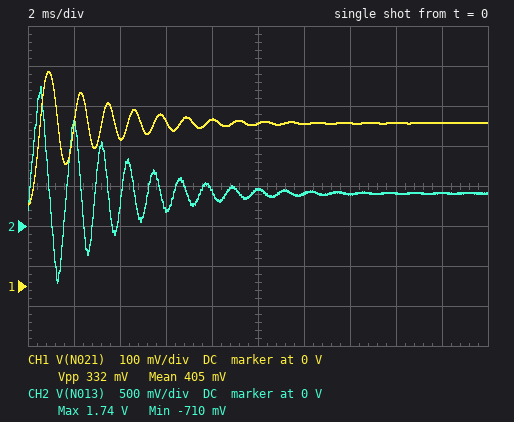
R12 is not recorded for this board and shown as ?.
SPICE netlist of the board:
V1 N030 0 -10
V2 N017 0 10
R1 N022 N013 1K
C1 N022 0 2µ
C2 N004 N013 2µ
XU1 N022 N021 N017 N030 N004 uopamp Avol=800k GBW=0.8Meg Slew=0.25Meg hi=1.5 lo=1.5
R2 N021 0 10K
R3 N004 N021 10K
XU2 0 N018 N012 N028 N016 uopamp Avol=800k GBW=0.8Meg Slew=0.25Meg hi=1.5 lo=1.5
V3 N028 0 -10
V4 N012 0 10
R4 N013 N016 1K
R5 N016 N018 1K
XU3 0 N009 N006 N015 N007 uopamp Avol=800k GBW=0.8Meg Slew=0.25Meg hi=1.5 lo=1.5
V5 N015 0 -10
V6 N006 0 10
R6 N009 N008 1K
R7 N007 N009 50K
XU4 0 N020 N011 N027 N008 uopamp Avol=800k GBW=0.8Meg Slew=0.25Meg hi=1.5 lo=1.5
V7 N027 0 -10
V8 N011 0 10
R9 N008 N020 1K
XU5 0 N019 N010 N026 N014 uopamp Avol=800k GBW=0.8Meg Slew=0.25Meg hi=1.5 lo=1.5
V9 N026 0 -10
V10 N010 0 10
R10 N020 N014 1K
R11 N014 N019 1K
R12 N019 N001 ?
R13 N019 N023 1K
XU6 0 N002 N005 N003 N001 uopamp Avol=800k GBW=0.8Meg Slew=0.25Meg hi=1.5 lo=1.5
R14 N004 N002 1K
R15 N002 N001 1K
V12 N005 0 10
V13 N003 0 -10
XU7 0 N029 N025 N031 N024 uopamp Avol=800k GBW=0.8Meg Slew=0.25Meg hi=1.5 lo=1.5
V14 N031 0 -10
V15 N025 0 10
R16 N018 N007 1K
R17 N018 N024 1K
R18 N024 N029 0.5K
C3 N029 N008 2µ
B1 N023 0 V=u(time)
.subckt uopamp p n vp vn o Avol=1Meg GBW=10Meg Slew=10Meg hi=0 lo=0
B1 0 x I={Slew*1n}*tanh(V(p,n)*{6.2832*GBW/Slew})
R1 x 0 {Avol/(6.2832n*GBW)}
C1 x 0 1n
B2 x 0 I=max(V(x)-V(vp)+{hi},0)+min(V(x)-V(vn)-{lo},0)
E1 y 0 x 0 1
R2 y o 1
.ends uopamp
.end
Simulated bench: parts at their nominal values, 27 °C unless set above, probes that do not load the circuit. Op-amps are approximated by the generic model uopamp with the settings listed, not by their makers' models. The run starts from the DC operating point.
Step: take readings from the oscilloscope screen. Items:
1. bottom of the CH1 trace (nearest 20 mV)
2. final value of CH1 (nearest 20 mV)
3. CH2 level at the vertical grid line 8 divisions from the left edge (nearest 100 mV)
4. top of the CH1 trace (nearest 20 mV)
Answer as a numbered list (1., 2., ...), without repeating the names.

1. 200 mV
2. 400 mV
3. 400 mV
4. 540 mV
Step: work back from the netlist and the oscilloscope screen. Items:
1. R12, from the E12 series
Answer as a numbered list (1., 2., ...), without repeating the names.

1. 820 Ω
